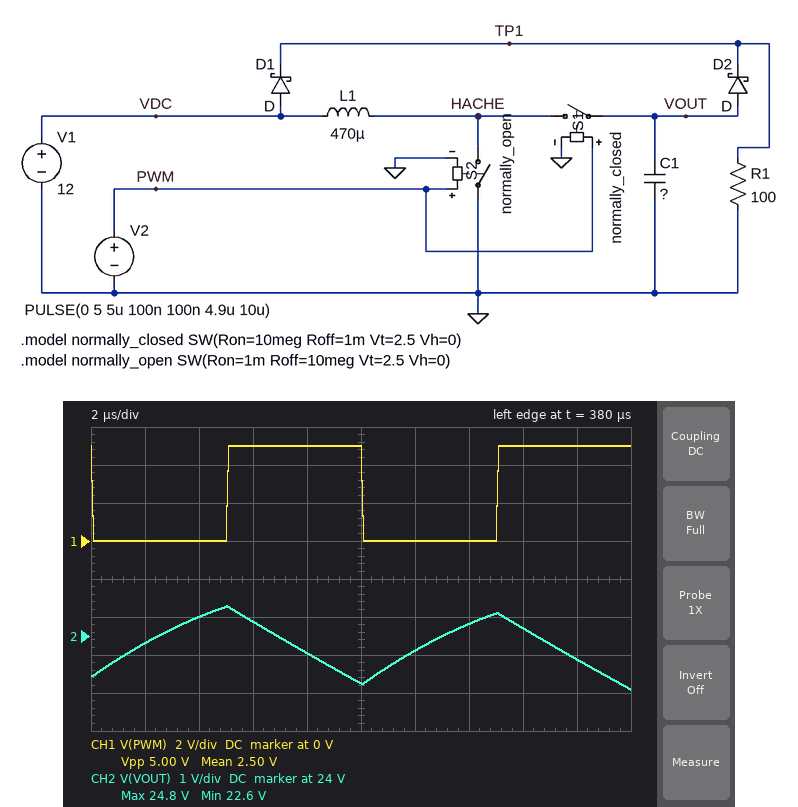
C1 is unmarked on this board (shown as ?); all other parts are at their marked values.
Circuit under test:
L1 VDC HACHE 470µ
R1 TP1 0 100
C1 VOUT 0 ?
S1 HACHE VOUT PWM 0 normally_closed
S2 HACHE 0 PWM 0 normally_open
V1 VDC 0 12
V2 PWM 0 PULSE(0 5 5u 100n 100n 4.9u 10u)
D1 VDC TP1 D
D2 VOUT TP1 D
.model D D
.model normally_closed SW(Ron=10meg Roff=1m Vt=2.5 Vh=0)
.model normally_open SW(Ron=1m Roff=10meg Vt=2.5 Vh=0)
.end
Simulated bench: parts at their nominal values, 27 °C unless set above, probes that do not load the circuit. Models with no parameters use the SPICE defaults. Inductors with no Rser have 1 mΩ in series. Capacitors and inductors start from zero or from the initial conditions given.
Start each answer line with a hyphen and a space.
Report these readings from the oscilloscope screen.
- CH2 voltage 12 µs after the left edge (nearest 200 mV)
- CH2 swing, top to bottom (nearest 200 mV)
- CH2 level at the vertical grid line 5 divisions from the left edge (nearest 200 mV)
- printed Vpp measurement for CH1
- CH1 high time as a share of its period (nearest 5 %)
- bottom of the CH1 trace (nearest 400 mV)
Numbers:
- 23.6 V
- 2.2 V
- 22.8 V
- 5.00 V
- 50 %
- 0 V
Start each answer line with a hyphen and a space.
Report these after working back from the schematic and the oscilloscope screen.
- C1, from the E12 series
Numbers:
- 560 nF
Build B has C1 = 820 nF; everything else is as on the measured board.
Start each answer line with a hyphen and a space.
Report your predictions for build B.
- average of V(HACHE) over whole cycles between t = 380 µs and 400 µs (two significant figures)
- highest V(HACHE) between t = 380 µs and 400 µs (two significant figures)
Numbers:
- 13 V
- 27 V
